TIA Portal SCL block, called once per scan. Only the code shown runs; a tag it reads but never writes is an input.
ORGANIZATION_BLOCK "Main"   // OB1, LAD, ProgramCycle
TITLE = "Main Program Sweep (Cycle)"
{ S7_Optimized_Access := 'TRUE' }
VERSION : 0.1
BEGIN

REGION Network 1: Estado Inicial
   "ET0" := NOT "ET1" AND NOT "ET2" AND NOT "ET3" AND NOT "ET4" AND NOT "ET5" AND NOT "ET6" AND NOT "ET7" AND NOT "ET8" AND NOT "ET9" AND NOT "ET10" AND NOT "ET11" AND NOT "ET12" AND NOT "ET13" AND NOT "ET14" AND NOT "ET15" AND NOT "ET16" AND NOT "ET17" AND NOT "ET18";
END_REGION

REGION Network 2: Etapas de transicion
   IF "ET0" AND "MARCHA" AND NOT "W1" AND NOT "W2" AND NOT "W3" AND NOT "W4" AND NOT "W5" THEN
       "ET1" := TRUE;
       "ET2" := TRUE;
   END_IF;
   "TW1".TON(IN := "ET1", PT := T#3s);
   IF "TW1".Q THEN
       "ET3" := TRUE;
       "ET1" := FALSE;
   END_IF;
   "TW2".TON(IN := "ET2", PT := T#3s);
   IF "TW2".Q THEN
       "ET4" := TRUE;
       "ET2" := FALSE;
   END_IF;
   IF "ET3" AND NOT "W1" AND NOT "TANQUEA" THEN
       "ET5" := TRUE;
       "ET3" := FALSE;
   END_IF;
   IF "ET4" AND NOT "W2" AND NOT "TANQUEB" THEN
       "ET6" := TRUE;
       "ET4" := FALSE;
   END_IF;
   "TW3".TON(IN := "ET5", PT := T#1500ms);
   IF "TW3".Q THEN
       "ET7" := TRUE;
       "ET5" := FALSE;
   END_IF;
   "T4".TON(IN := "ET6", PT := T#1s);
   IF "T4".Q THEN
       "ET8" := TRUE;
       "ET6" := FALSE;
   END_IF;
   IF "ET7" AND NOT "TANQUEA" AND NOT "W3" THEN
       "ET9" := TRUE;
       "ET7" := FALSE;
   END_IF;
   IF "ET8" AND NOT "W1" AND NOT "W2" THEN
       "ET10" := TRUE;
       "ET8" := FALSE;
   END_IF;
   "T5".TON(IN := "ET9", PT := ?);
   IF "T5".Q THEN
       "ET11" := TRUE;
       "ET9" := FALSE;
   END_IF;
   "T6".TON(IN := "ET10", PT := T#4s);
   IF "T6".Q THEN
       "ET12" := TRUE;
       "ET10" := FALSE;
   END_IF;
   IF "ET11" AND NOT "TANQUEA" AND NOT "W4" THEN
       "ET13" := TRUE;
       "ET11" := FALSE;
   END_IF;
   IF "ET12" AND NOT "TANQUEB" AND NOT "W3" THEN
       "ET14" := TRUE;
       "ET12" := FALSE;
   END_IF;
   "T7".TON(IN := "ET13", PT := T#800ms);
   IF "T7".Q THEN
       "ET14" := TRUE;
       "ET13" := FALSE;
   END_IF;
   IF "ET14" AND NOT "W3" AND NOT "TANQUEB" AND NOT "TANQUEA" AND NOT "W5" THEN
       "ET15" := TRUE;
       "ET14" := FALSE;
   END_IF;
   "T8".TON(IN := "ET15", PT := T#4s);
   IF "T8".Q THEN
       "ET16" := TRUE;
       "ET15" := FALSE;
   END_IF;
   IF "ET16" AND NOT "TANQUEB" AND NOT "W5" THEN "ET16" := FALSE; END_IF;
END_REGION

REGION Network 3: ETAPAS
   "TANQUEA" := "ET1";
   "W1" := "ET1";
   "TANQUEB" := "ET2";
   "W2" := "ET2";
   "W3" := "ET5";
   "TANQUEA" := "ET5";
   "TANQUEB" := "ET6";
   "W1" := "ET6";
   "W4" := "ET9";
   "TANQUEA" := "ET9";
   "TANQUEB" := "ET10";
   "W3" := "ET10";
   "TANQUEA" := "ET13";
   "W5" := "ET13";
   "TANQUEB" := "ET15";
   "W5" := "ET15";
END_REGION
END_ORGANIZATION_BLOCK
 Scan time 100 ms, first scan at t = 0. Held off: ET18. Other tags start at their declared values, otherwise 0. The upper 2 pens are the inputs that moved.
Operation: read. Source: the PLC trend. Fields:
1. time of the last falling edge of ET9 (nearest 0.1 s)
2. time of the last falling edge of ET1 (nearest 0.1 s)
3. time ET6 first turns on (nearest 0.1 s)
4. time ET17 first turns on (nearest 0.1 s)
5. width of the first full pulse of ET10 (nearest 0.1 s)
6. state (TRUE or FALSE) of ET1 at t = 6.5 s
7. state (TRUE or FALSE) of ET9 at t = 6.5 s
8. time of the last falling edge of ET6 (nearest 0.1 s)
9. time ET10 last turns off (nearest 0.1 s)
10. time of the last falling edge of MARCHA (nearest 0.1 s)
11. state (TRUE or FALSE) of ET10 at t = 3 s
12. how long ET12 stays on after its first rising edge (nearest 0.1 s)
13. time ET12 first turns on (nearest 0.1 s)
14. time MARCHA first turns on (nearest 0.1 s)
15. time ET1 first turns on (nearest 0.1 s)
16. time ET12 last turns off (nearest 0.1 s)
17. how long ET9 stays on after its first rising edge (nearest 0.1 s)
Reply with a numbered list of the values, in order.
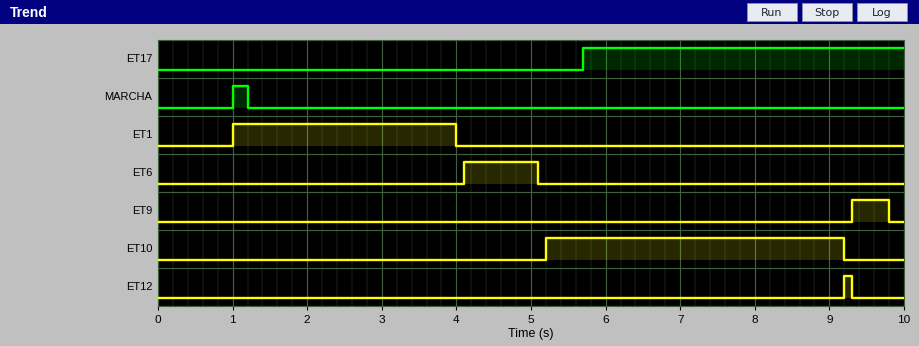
1. 9.8 s
2. 4.0 s
3. 4.1 s
4. 5.7 s
5. 4.0 s
6. FALSE
7. FALSE
8. 5.1 s
9. 9.2 s
10. 1.2 s
11. FALSE
12. 0.1 s
13. 9.2 s
14. 1.0 s
15. 1.0 s
16. 9.3 s
17. 0.5 s
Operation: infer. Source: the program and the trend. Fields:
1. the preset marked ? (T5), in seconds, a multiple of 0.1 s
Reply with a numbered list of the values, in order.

1. 0.5 s
